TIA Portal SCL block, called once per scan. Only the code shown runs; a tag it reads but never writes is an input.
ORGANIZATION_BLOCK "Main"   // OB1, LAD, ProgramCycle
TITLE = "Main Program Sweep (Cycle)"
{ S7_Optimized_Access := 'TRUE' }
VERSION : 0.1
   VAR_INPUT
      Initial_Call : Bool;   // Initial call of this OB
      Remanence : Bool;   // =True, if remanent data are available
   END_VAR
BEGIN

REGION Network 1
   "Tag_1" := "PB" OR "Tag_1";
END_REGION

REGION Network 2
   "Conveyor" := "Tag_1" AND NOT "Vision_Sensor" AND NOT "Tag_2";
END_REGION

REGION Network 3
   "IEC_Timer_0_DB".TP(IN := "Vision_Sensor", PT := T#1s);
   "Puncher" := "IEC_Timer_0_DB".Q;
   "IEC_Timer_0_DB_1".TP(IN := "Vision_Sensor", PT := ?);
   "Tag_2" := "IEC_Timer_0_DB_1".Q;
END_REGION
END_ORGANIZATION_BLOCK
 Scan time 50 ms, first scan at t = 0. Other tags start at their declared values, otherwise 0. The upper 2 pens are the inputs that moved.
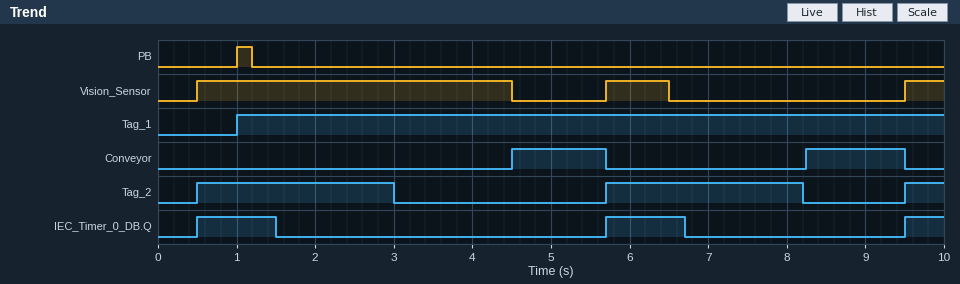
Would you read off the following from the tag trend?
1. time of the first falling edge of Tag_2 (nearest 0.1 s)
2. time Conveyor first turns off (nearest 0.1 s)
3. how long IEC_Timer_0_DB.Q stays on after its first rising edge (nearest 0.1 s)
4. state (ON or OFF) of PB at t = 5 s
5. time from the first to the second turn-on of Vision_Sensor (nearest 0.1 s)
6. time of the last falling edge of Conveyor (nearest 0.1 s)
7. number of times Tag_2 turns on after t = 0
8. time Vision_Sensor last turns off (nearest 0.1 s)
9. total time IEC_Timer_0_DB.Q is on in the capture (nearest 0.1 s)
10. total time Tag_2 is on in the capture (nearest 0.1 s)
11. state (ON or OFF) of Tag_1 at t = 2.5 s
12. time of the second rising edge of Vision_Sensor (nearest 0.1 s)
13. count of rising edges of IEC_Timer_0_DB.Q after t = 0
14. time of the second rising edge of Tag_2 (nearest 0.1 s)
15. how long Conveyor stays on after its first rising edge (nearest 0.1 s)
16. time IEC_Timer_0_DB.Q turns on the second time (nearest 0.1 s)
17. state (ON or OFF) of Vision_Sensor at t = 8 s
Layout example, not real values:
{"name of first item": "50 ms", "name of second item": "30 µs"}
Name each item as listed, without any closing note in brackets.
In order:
{"time of the first falling edge of Tag_2": "3.0 s", "time Conveyor first turns off": "5.7 s", "how long IEC_Timer_0_DB.Q stays on after its first rising edge": "1.0 s", "state (ON or OFF) of PB at t = 5 s": "OFF", "time from the first to the second turn-on of Vision_Sensor": "5.2 s", "time of the last falling edge of Conveyor": "9.5 s", "number of times Tag_2 turns on after t = 0": "3", "time Vision_Sensor last turns off": "6.5 s", "total time IEC_Timer_0_DB.Q is on in the capture": "2.5 s", "total time Tag_2 is on in the capture": "5.5 s", "state (ON or OFF) of Tag_1 at t = 2.5 s": "ON", "time of the second rising edge of Vision_Sensor": "5.7 s", "count of rising edges of IEC_Timer_0_DB.Q after t = 0": "3", "time of the second rising edge of Tag_2": "5.7 s", "how long Conveyor stays on after its first rising edge": "1.2 s", "time IEC_Timer_0_DB.Q turns on the second time": "5.7 s", "state (ON or OFF) of Vision_Sensor at t = 8 s": "OFF"}
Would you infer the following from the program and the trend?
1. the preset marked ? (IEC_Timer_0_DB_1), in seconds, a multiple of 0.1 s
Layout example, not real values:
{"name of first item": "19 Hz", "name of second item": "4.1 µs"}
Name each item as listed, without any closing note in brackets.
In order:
{"the preset marked ? (IEC_Timer_0_DB_1), in seconds, a multiple of 0.1 s": "2.5 s"}
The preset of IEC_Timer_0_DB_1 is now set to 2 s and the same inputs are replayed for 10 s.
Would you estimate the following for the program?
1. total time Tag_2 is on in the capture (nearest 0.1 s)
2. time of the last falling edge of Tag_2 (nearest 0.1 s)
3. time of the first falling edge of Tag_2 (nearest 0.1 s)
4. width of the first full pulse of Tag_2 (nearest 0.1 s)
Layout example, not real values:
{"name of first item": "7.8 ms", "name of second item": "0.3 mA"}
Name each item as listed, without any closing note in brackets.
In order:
{"total time Tag_2 is on in the capture": "4.5 s", "time of the last falling edge of Tag_2": "7.7 s", "time of the first falling edge of Tag_2": "2.5 s", "width of the first full pulse of Tag_2": "2.0 s"}
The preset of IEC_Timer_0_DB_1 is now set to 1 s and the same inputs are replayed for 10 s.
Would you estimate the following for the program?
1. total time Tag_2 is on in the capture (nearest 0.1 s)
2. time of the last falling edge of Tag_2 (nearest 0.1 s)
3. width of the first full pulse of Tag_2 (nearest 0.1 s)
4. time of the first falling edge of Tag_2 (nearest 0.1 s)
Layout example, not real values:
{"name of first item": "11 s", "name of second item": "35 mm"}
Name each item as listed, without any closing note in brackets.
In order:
{"total time Tag_2 is on in the capture": "2.5 s", "time of the last falling edge of Tag_2": "6.7 s", "width of the first full pulse of Tag_2": "1.0 s", "time of the first falling edge of Tag_2": "1.5 s"}
